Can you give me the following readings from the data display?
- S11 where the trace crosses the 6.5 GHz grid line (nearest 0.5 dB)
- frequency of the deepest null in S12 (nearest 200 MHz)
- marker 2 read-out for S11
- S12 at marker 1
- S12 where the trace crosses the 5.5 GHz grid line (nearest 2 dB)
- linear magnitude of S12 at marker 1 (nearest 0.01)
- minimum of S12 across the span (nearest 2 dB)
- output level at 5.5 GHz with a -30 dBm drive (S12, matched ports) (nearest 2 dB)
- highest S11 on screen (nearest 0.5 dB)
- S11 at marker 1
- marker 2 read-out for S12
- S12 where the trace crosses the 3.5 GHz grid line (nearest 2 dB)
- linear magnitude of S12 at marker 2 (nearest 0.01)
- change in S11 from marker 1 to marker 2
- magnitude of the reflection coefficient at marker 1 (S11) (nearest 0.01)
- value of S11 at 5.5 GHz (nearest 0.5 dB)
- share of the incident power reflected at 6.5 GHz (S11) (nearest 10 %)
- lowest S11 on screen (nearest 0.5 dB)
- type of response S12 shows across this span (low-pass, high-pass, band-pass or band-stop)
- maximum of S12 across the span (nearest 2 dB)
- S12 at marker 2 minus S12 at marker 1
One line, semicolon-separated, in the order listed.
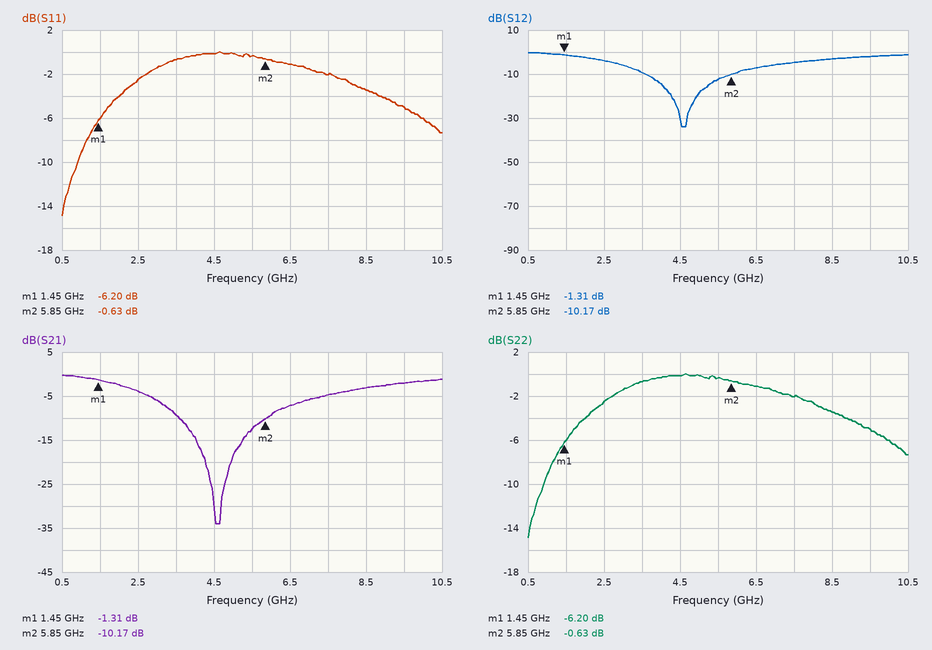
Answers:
-1.0 dB; 4.6 GHz; -0.63 dB; -1.31 dB; -12 dB; 0.86; -34 dB; -42 dBm; 0.0 dB; -6.20 dB; -10.17 dB; -10 dB; 0.31; 5.57 dB; 0.49; -0.5 dB; 80 %; -15.0 dB; band-stop; 0 dB; -8.86 dB
